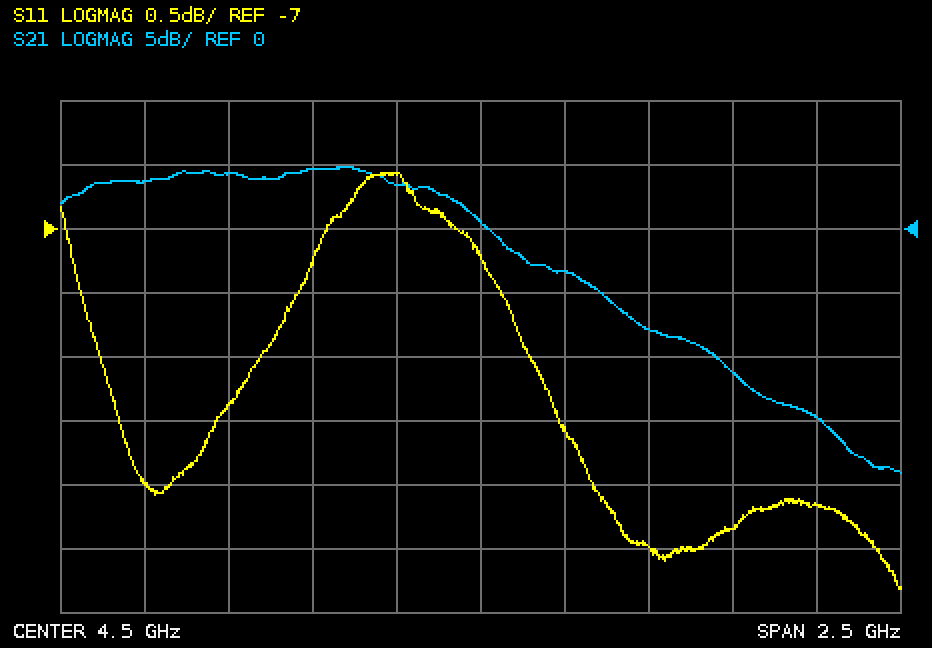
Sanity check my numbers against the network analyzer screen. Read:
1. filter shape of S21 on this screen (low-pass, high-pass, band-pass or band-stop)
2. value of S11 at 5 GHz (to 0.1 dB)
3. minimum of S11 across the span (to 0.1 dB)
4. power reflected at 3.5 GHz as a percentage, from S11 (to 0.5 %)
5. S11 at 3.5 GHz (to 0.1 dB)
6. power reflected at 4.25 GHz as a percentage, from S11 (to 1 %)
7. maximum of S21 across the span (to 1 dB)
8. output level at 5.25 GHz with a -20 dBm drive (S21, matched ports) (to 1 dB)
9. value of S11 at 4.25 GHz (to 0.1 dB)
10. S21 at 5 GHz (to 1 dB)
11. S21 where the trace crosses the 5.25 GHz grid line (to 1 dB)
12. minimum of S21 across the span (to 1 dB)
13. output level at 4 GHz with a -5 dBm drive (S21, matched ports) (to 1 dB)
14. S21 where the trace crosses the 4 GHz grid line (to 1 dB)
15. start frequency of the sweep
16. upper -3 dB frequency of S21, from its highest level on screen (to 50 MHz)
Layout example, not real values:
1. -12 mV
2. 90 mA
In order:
1. low-pass
2. -9.5 dB
3. -9.8 dB
4. 12.5 %
5. -9.0 dB
6. 22 %
7. 5 dB
8. -31 dBm
9. -6.6 dB
10. -8 dB
11. -11 dB
12. -19 dB
13. 0 dBm
14. 5 dB
15. 3.25 GHz
16. 4.45 GHz
